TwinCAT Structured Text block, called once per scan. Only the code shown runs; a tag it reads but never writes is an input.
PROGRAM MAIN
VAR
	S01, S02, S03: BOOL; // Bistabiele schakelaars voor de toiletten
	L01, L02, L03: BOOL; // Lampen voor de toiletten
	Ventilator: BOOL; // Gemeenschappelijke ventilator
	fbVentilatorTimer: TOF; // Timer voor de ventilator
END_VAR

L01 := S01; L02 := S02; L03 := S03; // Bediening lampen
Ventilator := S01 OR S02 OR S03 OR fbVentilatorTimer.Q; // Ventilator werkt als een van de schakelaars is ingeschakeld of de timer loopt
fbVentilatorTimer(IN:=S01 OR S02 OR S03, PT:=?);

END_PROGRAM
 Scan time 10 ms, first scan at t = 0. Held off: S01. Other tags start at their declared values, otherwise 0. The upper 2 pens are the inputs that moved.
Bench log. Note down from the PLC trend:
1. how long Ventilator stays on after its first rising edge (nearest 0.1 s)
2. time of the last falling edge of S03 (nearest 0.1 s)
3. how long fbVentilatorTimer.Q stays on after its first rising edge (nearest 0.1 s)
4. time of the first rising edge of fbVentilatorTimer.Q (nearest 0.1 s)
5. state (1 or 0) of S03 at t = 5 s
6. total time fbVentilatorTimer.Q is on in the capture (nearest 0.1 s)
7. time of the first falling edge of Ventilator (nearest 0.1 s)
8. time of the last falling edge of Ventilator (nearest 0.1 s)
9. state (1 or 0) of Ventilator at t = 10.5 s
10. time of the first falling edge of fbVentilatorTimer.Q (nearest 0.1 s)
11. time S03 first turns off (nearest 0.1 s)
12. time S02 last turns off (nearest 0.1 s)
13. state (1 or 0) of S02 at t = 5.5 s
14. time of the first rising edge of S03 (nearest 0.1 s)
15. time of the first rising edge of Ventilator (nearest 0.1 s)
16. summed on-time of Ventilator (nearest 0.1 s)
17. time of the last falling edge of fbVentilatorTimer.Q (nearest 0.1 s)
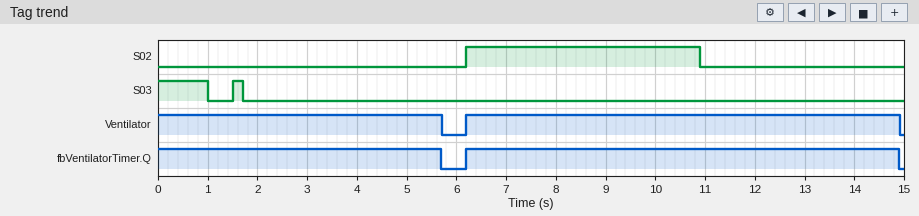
8.7 s
1.7 s
8.7 s
6.2 s
0
14.4 s
5.7 s
14.9 s
1
5.7 s
1.0 s
10.9 s
0
1.5 s
6.2 s
14.4 s
14.9 s
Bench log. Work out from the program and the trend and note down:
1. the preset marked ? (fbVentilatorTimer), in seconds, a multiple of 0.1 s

4.0 s
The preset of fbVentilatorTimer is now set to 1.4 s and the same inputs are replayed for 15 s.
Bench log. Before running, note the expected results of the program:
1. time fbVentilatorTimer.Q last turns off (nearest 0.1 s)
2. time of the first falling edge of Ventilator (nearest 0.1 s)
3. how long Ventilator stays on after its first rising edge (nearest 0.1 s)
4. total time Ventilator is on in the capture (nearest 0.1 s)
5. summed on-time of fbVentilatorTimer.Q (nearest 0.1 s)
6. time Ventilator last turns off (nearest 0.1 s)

12.3 s
3.1 s
6.1 s
9.2 s
9.2 s
12.3 s
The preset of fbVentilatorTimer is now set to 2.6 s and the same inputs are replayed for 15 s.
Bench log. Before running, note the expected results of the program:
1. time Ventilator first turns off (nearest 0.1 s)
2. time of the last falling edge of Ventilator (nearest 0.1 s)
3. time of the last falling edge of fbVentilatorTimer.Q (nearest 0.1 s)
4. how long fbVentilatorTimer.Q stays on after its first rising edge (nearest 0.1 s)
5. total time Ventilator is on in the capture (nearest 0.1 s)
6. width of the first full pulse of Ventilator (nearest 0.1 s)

4.3 s
13.5 s
13.5 s
7.3 s
11.6 s
7.3 s
